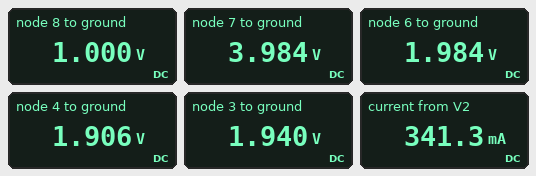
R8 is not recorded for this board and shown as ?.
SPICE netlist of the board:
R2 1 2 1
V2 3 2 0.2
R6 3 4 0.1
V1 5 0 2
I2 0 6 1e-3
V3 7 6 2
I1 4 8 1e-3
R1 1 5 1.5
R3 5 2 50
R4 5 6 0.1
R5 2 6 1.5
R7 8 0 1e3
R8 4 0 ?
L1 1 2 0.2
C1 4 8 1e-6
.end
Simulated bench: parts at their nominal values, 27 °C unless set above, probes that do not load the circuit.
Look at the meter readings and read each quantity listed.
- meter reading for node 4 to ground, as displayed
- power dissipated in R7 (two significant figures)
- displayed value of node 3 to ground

1.906 V
1.0 mW
1.940 V
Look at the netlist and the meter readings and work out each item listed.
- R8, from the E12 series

5.6 Ω
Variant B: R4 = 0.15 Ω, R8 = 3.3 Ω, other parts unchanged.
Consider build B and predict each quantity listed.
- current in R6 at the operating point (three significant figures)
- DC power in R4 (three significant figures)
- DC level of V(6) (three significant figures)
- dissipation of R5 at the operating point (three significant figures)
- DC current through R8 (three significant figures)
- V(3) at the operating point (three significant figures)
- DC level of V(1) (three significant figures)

528 mA
9.12 mW
1.96 V
91.9 mW
527 mA
1.79 V
1.59 V
